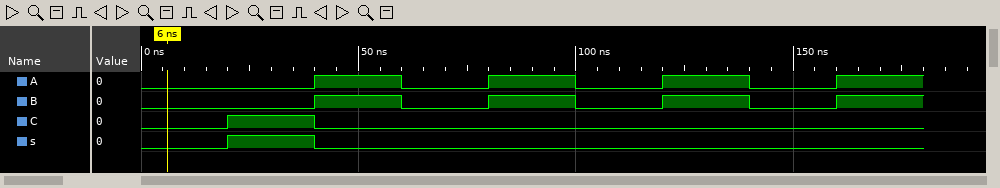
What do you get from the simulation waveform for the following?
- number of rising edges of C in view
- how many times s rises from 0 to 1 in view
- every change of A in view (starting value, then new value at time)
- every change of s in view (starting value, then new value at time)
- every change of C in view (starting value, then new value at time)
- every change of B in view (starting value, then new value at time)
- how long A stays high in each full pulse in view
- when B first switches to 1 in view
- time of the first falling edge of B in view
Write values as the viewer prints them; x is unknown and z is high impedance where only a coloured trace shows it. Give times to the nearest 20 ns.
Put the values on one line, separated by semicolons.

1; 1; 0, 1 at 40 ns, 0 at 60 ns, 1 at 80 ns, 0 at 100 ns, 1 at 120 ns, 0 at 140 ns, 1 at 160 ns; 0, 1 at 20 ns, 0 at 40 ns; 0, 1 at 20 ns, 0 at 40 ns; 0, 1 at 40 ns, 0 at 60 ns, 1 at 80 ns, 0 at 100 ns, 1 at 120 ns, 0 at 140 ns, 1 at 160 ns; 20 ns, 20 ns, 20 ns; 40 ns; 60 ns
